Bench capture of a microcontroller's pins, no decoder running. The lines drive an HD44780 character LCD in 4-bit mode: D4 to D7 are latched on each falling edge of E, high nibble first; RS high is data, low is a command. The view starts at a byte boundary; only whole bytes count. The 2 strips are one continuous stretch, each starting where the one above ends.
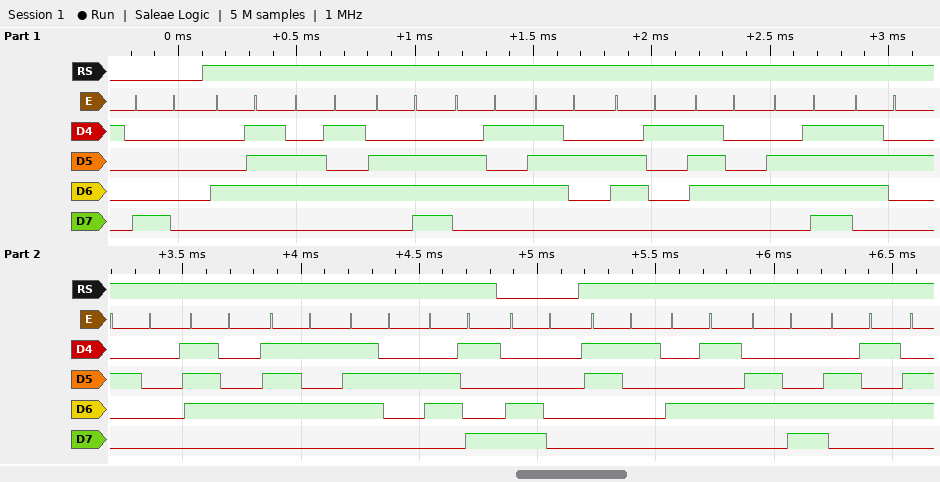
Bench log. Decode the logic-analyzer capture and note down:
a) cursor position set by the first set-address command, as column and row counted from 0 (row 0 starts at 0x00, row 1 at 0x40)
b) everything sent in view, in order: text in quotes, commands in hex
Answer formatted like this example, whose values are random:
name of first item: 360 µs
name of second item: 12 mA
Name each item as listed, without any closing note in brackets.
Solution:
cursor position set by the first set-address command, as column and row counted from 0: column 0, row 0
everything sent in view, in order: text in quotes, commands in hex: 0x80 "Generator turi" 0xC0 "1Ele"
